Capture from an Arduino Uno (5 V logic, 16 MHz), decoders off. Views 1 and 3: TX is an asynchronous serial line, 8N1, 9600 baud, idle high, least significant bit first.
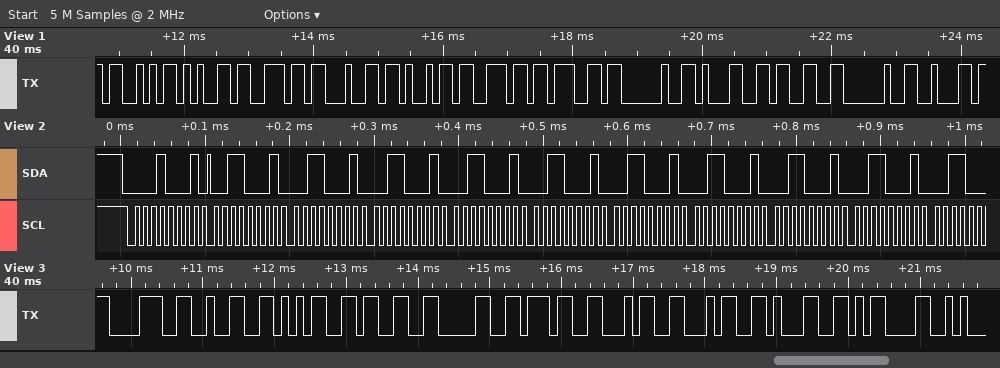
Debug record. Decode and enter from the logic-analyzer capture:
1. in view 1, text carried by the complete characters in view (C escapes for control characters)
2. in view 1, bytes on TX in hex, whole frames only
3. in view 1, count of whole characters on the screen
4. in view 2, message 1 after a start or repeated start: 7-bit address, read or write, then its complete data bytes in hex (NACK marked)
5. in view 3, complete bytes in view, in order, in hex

"Sending 13 b"
53 65 6E 64 69 6E 67 20 31 33 20 62
12
0x08 read: 31 31 31 31 31 31 31 31 31
38 32 35 33 30 37 34 34 31 0D
